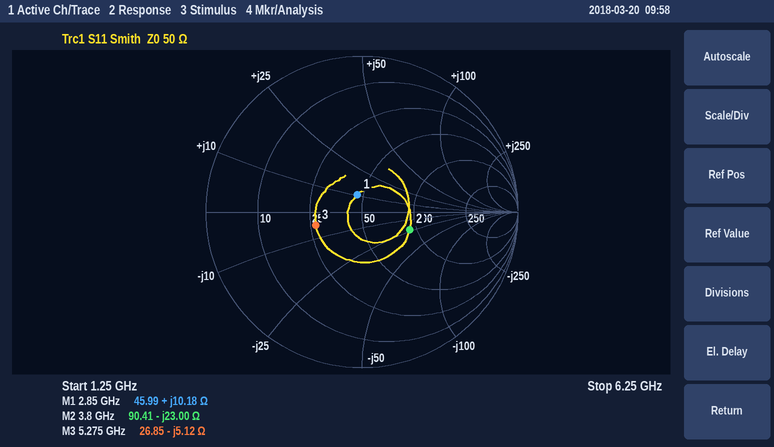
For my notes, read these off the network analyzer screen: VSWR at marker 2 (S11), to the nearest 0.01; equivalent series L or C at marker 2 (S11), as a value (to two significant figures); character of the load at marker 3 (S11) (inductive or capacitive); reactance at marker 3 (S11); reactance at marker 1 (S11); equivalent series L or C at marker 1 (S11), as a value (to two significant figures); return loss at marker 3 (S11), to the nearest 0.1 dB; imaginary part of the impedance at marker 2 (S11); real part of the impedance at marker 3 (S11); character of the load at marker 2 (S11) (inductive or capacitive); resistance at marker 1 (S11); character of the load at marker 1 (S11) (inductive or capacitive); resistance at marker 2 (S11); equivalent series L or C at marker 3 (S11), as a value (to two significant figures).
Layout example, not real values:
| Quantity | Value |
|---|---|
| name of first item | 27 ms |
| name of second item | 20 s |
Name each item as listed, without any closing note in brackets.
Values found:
| Quantity | Value |
|---|---|
| VSWR at marker 2 (S11), to the nearest 0.01 | 1.97 |
| equivalent series L or C at marker 2 (S11), as a value | 1.8 pF |
| character of the load at marker 3 (S11) | capacitive |
| reactance at marker 3 | -5.12 Ω |
| reactance at marker 1 | +10.18 Ω |
| equivalent series L or C at marker 1 (S11), as a value | 570 pH |
| return loss at marker 3 (S11), to the nearest 0.1 dB | 10.2 dB |
| imaginary part of the impedance at marker 2 | -23.00 Ω |
| real part of the impedance at marker 3 | 26.85 Ω |
| character of the load at marker 2 (S11) | capacitive |
| resistance at marker 1 | 45.99 Ω |
| character of the load at marker 1 (S11) | inductive |
| resistance at marker 2 | 90.41 Ω |
| equivalent series L or C at marker 3 (S11), as a value | 5.9 pF |
